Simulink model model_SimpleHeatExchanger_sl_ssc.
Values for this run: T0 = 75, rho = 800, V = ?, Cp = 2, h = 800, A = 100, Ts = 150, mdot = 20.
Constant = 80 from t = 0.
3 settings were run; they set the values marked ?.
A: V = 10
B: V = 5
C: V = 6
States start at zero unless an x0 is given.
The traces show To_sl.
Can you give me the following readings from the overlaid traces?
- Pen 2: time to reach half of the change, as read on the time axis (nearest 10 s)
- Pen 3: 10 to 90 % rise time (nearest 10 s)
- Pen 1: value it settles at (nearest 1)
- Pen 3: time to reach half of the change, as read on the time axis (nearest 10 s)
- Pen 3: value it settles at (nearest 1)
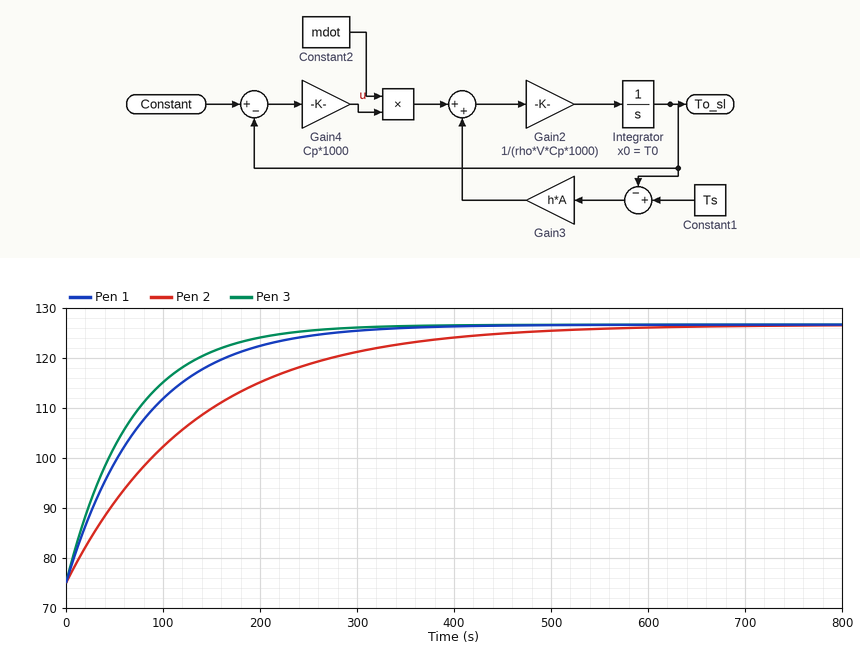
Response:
90 s
150 s
127
50 s
127
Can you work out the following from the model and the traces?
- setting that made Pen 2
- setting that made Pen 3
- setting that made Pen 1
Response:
A
B
C
